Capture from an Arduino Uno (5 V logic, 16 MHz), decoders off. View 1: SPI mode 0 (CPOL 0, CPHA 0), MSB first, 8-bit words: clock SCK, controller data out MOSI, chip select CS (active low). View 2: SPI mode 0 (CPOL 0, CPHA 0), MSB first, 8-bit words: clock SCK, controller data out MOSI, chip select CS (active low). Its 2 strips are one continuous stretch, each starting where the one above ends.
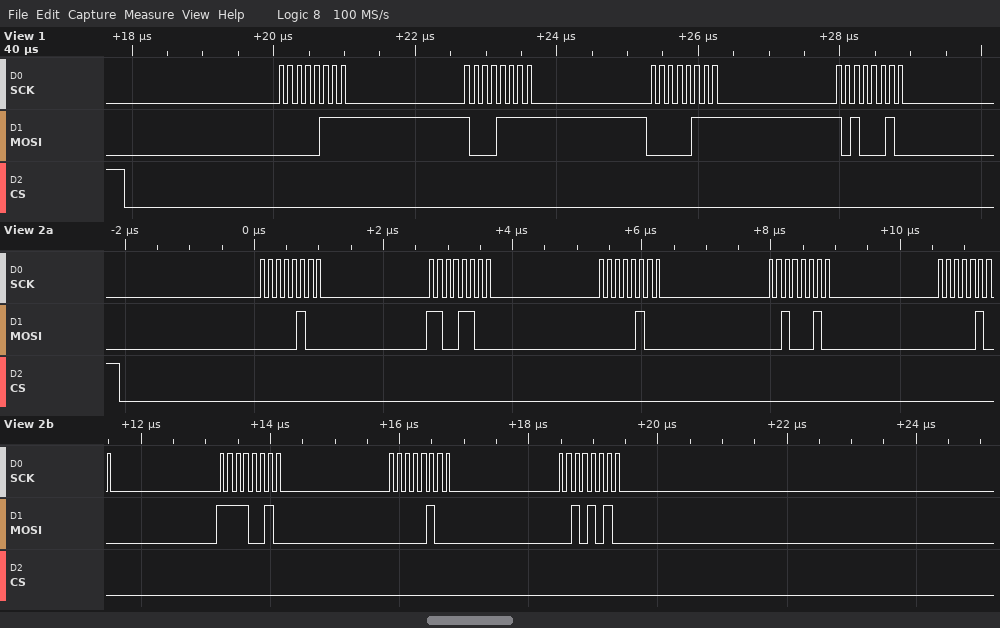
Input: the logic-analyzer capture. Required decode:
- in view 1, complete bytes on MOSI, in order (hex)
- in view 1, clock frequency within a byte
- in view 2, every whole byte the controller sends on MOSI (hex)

07 8F 07 A2
8 MHz
0x04 0xCC 0x04 0x22 0x04 0xF2 0x04 0x2A
